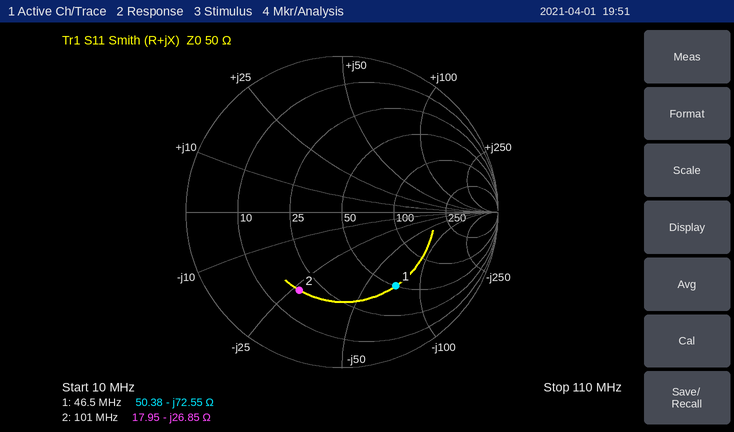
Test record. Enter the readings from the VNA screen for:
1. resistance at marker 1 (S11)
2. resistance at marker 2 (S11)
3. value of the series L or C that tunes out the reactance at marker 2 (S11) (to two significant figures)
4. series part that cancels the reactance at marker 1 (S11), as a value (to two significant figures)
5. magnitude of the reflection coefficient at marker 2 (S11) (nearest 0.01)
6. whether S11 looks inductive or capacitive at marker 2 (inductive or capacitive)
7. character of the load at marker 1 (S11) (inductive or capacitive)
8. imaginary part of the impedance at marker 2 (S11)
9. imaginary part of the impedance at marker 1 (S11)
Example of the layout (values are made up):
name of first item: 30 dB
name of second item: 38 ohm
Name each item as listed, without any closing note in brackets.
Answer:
resistance at marker 1: 50.38 Ω
resistance at marker 2: 17.95 Ω
value of the series L or C that tunes out the reactance at marker 2 (S11): 42 nH
series part that cancels the reactance at marker 1 (S11), as a value: 250 nH
magnitude of the reflection coefficient at marker 2 (S11): 0.57
whether S11 looks inductive or capacitive at marker 2: capacitive
character of the load at marker 1 (S11): capacitive
imaginary part of the impedance at marker 2: -26.85 Ω
imaginary part of the impedance at marker 1: -72.55 Ω
